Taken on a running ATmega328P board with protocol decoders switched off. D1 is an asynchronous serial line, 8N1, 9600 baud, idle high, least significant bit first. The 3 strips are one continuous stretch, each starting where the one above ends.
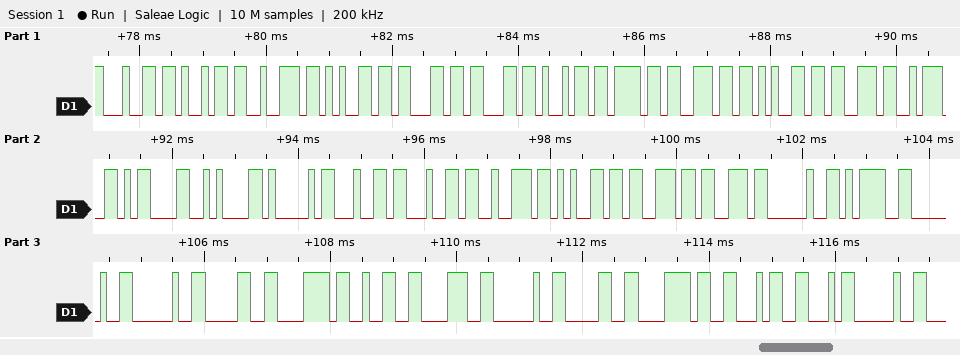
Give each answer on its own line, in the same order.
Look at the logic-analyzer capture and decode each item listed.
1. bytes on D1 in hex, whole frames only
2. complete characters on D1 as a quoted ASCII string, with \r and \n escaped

0x64 0x69 0x72 0x65 0x63 0x63 0x69 0x6F 0x6E 0x65 0x73 0x3A 0x0D 0x0A 0x41 0x64 0x64 0x72 0x65 0x73 0x73 0x20 0x3D 0x20 0x20 0x30 0x78 0x32 0x38 0x20 0x30 0x78 0x46 0x46 0x20
"direcciones:\r\nAddress =  0x28 0xFF "
